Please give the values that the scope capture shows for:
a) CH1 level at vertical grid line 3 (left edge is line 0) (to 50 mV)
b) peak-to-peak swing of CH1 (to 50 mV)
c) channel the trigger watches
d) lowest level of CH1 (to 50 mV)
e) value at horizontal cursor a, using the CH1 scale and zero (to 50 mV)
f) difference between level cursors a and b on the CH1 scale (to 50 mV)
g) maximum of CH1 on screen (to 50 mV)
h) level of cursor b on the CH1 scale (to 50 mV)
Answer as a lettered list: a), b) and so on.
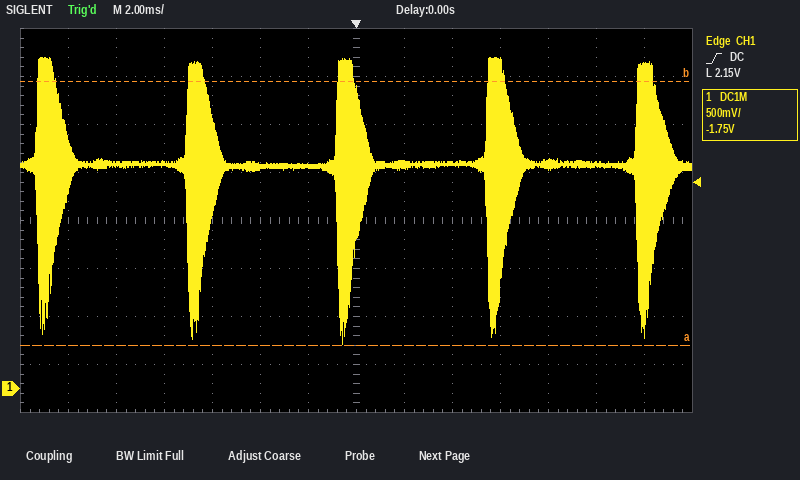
a) 2.35 V
b) 3.00 V
c) CH1
d) 450 mV
e) 450 mV
f) 2.75 V
g) 3.45 V
h) 3.20 V
